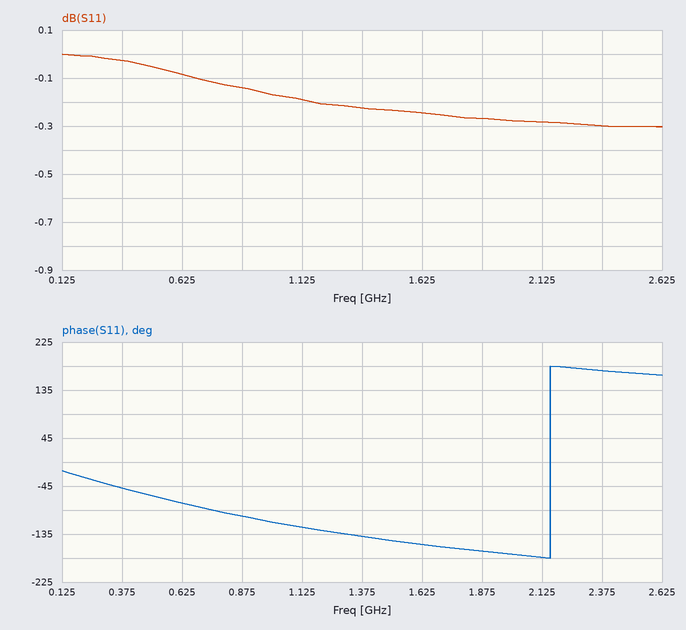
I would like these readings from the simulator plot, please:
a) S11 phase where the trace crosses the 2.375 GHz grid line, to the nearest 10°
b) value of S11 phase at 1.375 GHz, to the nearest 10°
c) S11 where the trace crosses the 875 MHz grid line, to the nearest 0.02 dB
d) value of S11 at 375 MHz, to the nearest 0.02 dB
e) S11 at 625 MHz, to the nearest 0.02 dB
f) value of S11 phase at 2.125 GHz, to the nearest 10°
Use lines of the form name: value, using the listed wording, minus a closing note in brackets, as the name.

S11 phase where the trace crosses the 2.375 GHz grid line, to the nearest 10°: 170°
value of S11 phase at 1.375 GHz, to the nearest 10°: -140°
S11 where the trace crosses the 875 MHz grid line, to the nearest 0.02 dB: -0.14 dB
value of S11 at 375 MHz, to the nearest 0.02 dB: -0.02 dB
S11 at 625 MHz, to the nearest 0.02 dB: -0.08 dB
value of S11 phase at 2.125 GHz, to the nearest 10°: -180°
